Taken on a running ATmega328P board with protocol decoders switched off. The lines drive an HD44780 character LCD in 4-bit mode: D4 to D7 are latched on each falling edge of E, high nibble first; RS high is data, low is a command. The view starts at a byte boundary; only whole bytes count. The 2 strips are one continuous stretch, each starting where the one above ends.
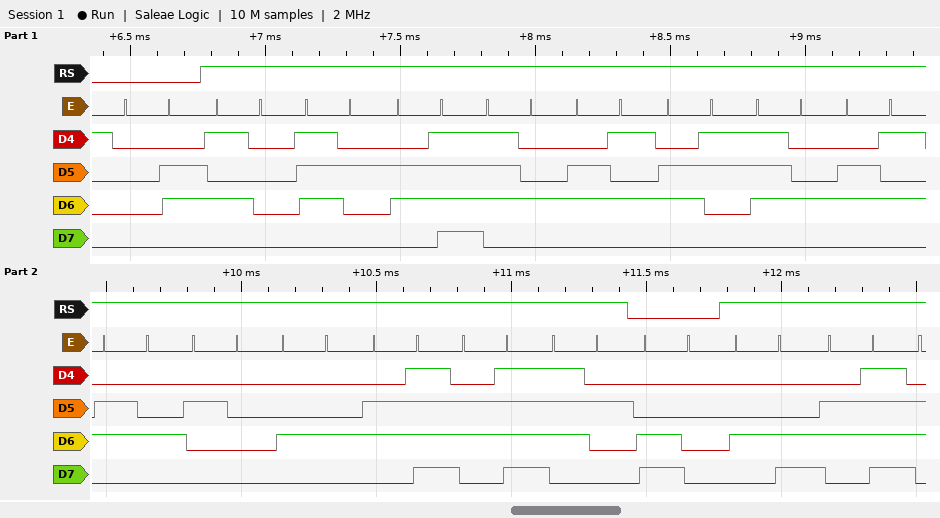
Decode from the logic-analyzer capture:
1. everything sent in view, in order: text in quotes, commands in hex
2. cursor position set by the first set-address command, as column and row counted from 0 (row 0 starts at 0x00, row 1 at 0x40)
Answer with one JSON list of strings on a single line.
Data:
["0x06 \"Protected Door\" 0xC0 \"Lo\"", "column 0, row 1"]
